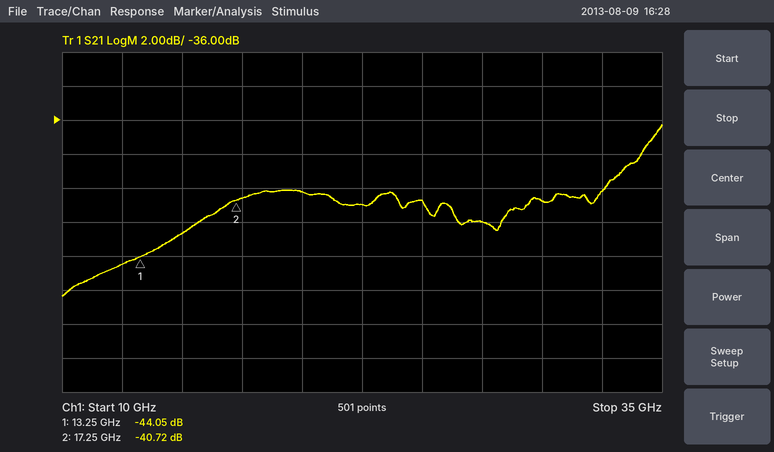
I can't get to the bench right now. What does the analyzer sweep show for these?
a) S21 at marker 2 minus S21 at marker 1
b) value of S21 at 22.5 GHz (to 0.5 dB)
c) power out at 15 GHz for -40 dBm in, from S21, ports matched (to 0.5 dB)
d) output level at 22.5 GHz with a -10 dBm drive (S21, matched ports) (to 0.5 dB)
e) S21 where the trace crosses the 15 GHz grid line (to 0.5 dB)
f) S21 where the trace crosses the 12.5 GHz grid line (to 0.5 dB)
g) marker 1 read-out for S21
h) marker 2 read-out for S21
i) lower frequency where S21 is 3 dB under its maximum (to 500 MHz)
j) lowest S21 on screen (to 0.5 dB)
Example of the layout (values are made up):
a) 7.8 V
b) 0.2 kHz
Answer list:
a) 3.33 dB
b) -41.0 dB
c) -82.5 dBm
d) -51.0 dBm
e) -42.5 dB
f) -44.5 dB
g) -44.05 dB
h) -40.72 dB
i) 33.0 GHz
j) -46.5 dB
